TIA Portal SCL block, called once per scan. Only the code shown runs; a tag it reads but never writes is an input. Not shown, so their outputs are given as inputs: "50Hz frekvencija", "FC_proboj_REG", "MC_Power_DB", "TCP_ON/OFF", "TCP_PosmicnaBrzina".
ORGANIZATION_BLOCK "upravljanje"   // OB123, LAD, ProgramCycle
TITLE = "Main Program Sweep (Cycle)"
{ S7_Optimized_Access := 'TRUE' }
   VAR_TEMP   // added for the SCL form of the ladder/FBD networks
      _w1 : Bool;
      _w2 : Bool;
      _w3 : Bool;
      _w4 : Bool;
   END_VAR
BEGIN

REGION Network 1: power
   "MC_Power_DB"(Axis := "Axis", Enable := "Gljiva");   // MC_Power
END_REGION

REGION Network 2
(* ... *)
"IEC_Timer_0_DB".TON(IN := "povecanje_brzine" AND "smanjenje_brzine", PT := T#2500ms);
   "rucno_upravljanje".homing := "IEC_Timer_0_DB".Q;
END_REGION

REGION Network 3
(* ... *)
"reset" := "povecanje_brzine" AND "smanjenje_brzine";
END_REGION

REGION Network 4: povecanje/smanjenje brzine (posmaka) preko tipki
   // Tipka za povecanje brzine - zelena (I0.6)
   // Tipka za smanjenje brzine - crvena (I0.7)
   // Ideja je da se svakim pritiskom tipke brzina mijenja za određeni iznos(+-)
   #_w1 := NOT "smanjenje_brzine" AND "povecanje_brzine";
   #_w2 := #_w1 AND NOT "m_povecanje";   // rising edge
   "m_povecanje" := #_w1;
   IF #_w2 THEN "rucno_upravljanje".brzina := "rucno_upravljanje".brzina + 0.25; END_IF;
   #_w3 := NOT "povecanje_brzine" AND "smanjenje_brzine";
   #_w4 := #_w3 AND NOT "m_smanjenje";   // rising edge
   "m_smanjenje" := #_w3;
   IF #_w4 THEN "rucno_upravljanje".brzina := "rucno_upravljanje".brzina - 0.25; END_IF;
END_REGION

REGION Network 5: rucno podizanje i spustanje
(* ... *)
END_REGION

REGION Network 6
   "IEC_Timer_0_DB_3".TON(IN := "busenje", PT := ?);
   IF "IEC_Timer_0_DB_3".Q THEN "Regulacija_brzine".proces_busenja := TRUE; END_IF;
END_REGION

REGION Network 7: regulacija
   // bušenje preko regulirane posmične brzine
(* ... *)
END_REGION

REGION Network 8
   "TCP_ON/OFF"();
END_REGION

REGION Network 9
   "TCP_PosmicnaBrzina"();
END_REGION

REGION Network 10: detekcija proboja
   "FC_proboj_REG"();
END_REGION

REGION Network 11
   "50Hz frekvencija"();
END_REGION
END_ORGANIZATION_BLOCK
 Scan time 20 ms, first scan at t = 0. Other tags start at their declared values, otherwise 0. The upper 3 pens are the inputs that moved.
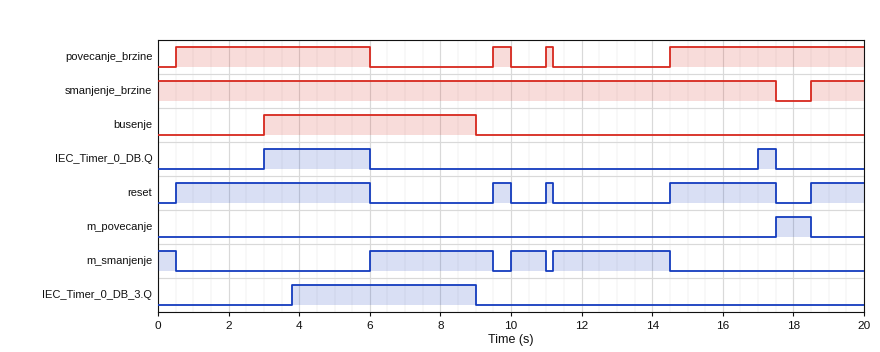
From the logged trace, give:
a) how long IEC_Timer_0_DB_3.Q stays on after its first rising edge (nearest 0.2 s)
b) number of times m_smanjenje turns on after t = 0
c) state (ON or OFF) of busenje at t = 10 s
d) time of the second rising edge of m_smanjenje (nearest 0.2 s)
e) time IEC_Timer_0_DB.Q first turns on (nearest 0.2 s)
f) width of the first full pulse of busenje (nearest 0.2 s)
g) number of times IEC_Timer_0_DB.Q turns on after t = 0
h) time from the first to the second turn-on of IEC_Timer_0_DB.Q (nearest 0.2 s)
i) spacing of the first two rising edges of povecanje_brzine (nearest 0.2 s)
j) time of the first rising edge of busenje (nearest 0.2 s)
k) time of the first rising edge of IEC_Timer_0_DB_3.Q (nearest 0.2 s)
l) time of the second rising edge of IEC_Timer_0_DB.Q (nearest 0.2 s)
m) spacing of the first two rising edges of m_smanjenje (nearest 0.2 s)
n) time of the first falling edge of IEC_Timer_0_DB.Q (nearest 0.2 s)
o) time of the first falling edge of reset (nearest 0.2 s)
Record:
5.2 s
3
OFF
10.0 s
3.0 s
6.0 s
2
14.0 s
9.0 s
3.0 s
3.8 s
17.0 s
4.0 s
6.0 s
6.0 s
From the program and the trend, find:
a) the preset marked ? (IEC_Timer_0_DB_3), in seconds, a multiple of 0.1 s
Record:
0.8 s
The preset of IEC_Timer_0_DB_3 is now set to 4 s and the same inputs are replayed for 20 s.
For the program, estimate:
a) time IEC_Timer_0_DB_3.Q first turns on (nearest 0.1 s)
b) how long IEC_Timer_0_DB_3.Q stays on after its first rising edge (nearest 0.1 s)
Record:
7.0 s
2.0 s
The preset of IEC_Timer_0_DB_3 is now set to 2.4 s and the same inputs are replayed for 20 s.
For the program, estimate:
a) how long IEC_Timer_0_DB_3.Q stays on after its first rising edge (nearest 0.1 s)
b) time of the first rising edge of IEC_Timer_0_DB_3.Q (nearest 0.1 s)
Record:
3.6 s
5.4 s
